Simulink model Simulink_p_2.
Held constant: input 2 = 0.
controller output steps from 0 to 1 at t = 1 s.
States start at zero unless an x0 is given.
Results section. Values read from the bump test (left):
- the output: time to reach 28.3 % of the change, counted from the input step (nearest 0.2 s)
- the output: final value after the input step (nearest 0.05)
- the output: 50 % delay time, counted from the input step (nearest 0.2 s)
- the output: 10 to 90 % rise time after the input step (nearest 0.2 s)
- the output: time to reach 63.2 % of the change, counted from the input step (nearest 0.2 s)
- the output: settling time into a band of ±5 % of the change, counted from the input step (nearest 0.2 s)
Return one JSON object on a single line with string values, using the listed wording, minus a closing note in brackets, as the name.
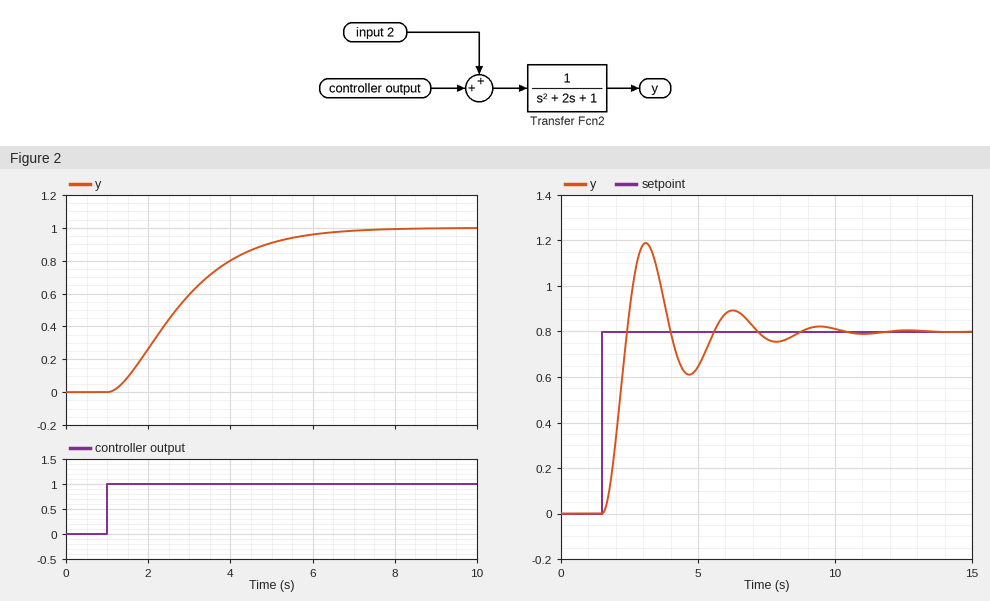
{"the output: time to reach 28.3 % of the change, counted from the input step": "1.0 s", "the output: final value after the input step": "1.00", "the output: 50 % delay time, counted from the input step": "1.6 s", "the output: 10 to 90 % rise time after the input step": "3.4 s", "the output: time to reach 63.2 % of the change, counted from the input step": "2.2 s", "the output: settling time into a band of ±5 % of the change, counted from the input step": "4.8 s"}
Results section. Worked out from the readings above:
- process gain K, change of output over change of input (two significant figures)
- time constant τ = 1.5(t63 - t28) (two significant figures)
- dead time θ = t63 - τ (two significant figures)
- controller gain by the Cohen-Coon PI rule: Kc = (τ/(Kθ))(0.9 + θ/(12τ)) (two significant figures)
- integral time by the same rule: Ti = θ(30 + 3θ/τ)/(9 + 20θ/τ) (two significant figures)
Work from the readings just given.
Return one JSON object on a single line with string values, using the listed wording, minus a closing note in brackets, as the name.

{"process gain K, change of output over change of input": "1.0", "time constant τ = 1.5(t63 - t28)": "1.8 s", "dead time θ = t63 - τ": "0.40 s", "controller gain by the Cohen-Coon PI rule: Kc = (τ/(Kθ))(0.9 + θ/(12τ))": "4.1", "integral time by the same rule: Ti = θ(30 + 3θ/τ)/(9 + 20θ/τ)": "0.91 s"}
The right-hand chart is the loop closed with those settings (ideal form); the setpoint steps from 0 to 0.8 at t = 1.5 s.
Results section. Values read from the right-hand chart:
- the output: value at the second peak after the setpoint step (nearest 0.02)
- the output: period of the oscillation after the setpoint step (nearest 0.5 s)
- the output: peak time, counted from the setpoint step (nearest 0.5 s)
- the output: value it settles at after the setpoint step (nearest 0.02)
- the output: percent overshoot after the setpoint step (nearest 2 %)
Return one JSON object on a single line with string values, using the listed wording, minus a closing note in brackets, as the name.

{"the output: value at the second peak after the setpoint step": "0.90", "the output: period of the oscillation after the setpoint step": "3.0 s", "the output: peak time, counted from the setpoint step": "1.5 s", "the output: value it settles at after the setpoint step": "0.80", "the output: percent overshoot after the setpoint step": "48 %"}
